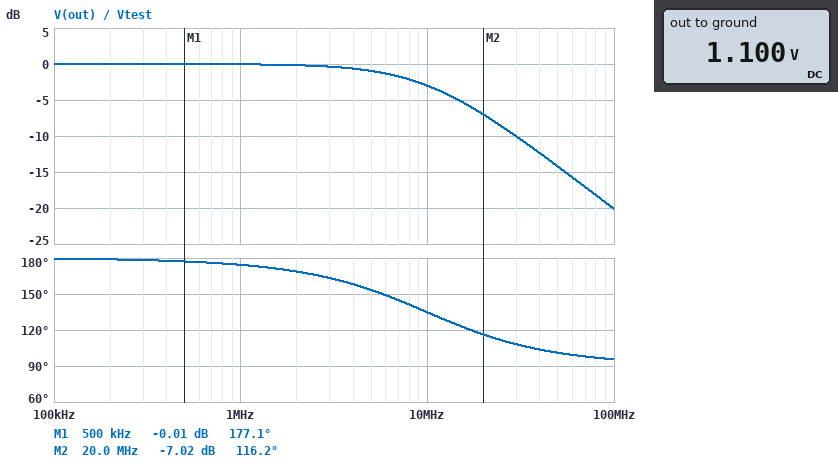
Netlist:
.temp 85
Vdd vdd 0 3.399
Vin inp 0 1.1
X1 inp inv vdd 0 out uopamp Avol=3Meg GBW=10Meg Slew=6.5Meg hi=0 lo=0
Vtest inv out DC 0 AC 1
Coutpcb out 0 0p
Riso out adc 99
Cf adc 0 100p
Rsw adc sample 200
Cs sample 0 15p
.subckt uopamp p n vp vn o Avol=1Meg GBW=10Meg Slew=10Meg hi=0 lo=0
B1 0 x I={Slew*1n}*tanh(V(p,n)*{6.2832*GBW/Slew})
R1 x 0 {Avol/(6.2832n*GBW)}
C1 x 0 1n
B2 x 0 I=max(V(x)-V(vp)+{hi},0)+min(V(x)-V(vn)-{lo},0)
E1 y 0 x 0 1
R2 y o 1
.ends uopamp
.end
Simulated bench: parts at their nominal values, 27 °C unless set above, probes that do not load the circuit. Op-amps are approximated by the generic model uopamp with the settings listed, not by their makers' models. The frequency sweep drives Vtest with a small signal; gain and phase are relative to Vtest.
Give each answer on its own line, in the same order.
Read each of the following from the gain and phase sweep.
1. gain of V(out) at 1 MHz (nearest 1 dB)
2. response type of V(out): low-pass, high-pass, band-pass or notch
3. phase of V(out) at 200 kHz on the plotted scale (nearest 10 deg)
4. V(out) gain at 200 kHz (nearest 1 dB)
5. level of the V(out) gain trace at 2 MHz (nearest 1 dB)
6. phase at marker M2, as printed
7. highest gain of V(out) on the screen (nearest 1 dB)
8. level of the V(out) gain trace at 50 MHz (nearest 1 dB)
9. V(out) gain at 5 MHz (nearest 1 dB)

0 dB
low-pass
180 deg
0 dB
0 dB
116.2 deg
0 dB
-14 dB
-1 dB
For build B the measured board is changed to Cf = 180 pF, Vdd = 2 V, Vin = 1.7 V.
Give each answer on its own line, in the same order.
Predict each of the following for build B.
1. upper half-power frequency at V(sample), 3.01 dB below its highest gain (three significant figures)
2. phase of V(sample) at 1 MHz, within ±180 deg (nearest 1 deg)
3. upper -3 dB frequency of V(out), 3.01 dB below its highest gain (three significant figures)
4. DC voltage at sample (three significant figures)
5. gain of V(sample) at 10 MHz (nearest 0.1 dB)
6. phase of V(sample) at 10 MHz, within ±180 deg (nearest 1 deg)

5.72 MHz
166 deg
9.99 MHz
1.70 V
-7.1 dB
74 deg
